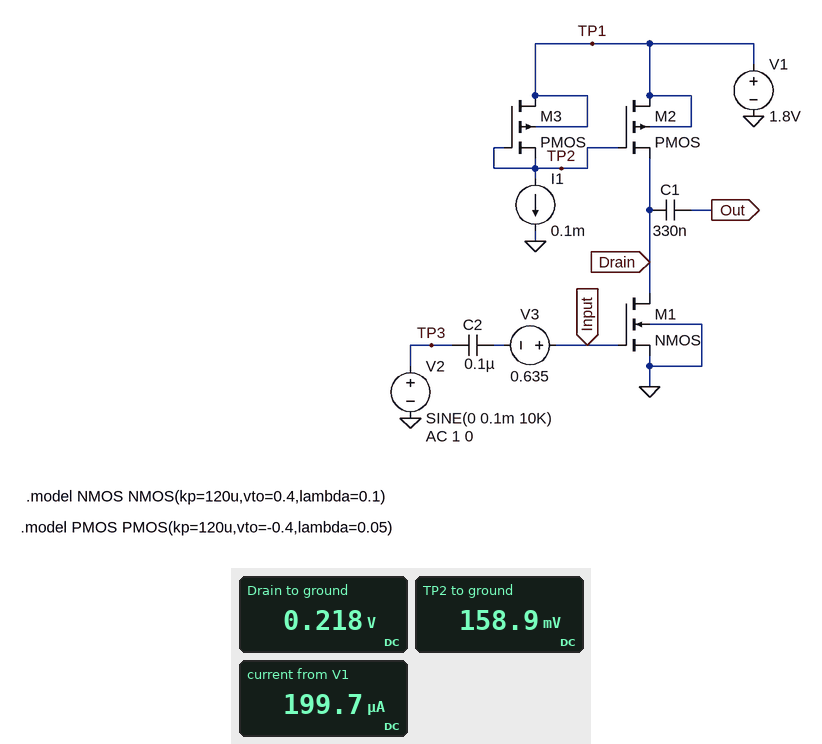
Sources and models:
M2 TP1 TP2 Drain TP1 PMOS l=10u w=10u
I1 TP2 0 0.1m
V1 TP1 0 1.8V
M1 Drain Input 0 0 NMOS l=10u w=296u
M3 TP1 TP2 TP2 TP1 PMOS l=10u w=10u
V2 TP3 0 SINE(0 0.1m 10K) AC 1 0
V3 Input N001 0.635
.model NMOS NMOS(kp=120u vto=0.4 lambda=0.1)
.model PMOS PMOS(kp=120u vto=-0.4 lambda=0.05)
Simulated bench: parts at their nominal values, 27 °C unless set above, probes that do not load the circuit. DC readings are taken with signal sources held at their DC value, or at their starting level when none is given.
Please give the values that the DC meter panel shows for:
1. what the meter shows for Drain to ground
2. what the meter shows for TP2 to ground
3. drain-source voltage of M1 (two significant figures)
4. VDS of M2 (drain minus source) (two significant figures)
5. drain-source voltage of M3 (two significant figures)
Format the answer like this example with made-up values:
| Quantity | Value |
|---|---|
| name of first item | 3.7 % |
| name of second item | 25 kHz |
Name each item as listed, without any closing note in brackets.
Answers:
| Quantity | Value |
|---|---|
| what the meter shows for Drain to ground | 0.218 V |
| what the meter shows for TP2 to ground | 158.9 mV |
| drain-source voltage of M1 | 220 mV |
| VDS of M2 (drain minus source) | 1.6 V |
| drain-source voltage of M3 | 1.6 V |
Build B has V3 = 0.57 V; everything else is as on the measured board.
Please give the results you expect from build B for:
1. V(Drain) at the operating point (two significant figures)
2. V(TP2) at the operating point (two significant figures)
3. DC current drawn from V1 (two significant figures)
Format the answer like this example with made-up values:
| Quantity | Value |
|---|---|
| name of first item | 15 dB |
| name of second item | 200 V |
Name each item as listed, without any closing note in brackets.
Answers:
| Quantity | Value |
|---|---|
| V(Drain) at the operating point | 1.3 V |
| V(TP2) at the operating point | 160 mV |
| DC current drawn from V1 | 160 µA |
